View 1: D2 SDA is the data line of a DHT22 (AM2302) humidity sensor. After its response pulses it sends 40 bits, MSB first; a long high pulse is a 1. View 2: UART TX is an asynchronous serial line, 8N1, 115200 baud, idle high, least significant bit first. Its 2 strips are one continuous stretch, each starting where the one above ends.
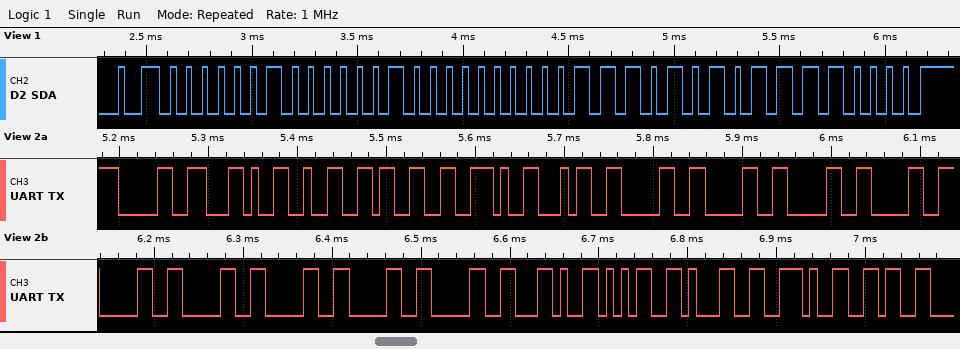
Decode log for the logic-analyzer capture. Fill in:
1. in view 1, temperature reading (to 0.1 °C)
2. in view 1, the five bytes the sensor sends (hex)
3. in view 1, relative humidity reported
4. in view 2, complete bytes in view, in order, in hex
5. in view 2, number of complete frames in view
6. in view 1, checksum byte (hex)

23.4 °C
02 04 00 EA F0
51.6 %
30 2C 32 33 2E 34 30 30 30 30 30 30 30 30 30 2C 35 31 2E 36
20
0xF0
